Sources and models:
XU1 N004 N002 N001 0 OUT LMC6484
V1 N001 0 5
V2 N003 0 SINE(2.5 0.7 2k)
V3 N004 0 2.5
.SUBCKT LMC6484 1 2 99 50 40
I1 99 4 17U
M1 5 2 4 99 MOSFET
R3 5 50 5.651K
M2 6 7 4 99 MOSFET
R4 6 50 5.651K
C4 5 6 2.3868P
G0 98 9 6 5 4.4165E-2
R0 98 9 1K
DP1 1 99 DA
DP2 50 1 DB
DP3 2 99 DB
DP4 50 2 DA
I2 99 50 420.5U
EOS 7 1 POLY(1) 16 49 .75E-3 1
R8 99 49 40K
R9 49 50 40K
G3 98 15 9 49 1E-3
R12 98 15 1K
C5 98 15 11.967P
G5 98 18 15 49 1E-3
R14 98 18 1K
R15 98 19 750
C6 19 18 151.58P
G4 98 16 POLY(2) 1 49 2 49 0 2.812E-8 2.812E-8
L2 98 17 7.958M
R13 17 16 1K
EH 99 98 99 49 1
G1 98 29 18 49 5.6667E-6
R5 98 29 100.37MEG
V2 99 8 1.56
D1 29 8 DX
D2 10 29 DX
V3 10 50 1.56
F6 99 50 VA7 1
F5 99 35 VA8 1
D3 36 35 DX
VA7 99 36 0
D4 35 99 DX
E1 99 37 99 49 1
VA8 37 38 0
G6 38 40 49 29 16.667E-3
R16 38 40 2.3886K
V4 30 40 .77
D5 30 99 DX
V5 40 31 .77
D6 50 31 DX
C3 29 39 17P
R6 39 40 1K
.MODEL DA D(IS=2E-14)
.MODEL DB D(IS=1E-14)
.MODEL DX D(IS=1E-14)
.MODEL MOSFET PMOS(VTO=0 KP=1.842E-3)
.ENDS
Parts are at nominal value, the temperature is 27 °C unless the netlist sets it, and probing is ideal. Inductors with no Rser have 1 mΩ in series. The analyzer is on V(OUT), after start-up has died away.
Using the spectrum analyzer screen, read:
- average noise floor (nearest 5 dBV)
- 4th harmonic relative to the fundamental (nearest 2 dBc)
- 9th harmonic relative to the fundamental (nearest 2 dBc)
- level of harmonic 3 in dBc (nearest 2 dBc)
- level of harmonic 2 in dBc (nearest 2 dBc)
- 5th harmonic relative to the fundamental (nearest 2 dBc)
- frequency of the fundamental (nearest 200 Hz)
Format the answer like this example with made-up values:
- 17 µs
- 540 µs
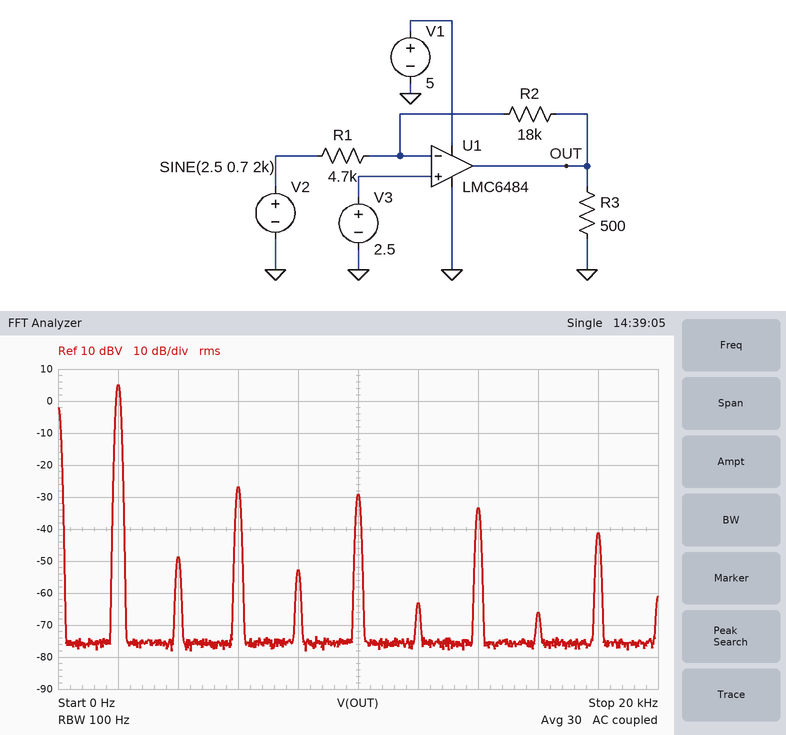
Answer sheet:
- -75 dBV
- -58 dBc
- -46 dBc
- -32 dBc
- -54 dBc
- -34 dBc
- 2.0 kHz
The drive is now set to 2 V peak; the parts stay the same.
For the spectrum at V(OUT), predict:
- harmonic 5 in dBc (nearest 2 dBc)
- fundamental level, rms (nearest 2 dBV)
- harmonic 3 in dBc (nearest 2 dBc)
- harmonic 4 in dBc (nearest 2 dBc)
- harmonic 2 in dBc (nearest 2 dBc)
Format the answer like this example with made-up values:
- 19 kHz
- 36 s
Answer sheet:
- -18 dBc
- 6 dBV
- -10 dBc
- -60 dBc
- -58 dBc
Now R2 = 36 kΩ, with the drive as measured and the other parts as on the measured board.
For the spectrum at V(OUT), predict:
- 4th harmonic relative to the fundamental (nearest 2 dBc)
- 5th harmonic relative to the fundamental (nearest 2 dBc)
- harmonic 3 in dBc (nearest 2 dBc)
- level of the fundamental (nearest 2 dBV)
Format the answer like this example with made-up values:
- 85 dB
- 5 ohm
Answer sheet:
- -56 dBc
- -24 dBc
- -12 dBc
- 6 dBV
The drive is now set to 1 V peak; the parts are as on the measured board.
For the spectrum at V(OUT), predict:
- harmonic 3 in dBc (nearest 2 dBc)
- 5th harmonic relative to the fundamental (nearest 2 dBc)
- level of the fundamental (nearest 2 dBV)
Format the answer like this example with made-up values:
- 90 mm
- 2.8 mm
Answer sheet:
- -16 dBc
- -40 dBc
- 6 dBV
